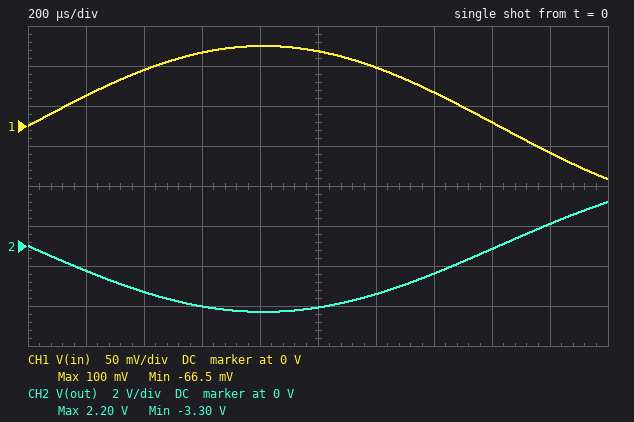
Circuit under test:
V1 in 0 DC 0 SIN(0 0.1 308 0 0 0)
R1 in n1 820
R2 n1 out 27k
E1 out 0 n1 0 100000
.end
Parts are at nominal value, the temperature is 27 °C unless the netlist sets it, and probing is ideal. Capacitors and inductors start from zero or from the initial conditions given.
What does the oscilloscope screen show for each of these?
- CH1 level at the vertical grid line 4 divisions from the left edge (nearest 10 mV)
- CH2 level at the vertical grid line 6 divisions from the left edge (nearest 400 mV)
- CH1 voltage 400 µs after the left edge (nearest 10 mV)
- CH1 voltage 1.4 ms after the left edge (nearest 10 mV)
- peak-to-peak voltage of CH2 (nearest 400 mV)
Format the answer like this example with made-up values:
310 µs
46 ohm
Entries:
100 mV
-2.4 V
70 mV
40 mV
5.6 V
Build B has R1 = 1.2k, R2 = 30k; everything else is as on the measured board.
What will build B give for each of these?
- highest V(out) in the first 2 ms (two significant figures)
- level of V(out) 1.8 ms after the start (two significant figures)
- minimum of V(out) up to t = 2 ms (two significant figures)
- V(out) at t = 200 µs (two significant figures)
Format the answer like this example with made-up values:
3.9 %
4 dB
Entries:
1.7 V
840 mV
-2.5 V
-940 mV
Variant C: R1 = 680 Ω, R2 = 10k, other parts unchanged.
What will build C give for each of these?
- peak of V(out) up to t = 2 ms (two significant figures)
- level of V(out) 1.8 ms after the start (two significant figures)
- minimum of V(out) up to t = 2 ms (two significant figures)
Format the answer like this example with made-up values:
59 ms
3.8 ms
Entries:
980 mV
490 mV
-1.5 V
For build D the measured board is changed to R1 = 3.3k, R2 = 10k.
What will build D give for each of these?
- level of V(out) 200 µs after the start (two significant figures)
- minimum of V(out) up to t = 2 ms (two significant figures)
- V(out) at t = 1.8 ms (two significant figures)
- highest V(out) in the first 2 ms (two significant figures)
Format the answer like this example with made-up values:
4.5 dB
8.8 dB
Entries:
-110 mV
-300 mV
100 mV
200 mV
